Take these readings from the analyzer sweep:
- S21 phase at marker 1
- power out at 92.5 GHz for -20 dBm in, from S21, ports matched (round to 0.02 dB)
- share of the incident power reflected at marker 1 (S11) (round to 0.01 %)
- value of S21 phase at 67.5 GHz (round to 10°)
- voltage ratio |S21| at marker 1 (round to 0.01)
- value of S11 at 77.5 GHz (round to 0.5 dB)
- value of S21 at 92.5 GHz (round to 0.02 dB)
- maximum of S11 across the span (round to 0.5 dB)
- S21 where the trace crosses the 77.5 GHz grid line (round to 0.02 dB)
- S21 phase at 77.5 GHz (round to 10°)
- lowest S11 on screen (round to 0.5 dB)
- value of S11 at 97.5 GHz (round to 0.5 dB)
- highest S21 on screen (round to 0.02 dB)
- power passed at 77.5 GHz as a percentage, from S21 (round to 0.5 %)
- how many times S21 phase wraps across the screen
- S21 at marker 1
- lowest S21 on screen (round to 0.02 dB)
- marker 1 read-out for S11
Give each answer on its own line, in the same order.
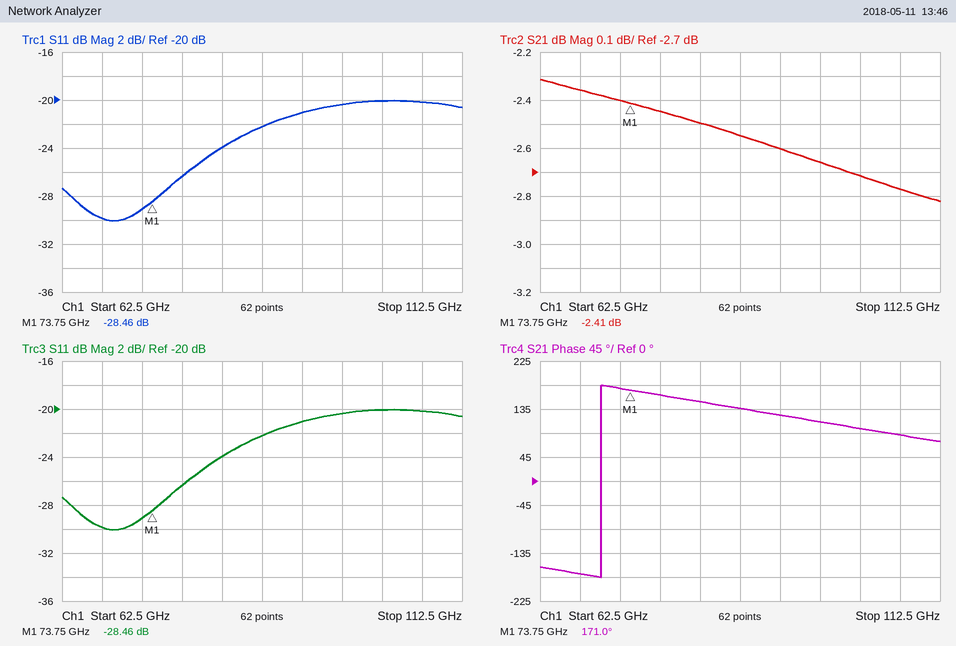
171.0°
-22.60 dBm
0.14 %
-170°
0.76
-26.5 dB
-2.60 dB
-20.0 dB
-2.44 dB
160°
-30.0 dB
-20.5 dB
-2.32 dB
57.0 %
1
-2.41 dB
-2.82 dB
-28.46 dB
